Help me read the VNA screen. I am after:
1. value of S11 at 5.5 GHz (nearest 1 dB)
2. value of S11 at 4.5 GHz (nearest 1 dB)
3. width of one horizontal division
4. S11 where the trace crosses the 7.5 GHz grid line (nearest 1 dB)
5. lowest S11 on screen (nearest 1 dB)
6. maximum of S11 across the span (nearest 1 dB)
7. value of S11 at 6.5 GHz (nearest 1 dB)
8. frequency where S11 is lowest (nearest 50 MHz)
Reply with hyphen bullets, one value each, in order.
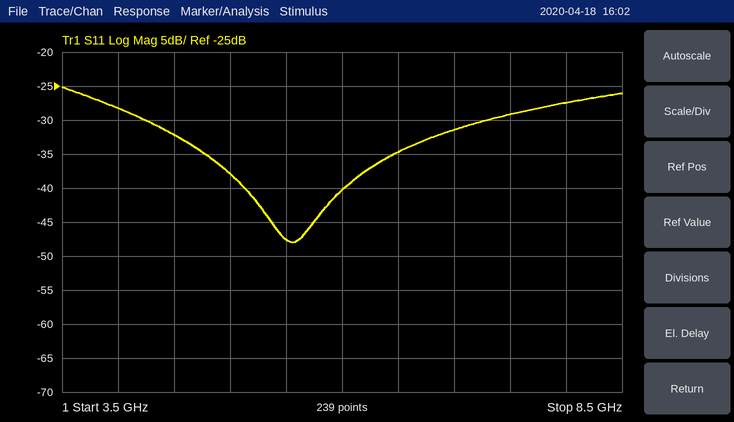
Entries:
- -48 dB
- -32 dB
- 500 MHz
- -29 dB
- -48 dB
- -25 dB
- -35 dB
- 5.55 GHz
